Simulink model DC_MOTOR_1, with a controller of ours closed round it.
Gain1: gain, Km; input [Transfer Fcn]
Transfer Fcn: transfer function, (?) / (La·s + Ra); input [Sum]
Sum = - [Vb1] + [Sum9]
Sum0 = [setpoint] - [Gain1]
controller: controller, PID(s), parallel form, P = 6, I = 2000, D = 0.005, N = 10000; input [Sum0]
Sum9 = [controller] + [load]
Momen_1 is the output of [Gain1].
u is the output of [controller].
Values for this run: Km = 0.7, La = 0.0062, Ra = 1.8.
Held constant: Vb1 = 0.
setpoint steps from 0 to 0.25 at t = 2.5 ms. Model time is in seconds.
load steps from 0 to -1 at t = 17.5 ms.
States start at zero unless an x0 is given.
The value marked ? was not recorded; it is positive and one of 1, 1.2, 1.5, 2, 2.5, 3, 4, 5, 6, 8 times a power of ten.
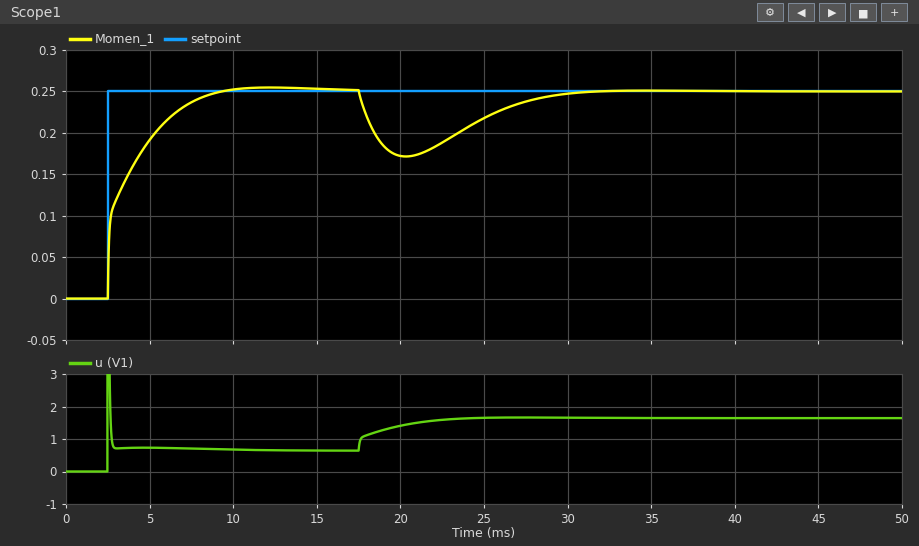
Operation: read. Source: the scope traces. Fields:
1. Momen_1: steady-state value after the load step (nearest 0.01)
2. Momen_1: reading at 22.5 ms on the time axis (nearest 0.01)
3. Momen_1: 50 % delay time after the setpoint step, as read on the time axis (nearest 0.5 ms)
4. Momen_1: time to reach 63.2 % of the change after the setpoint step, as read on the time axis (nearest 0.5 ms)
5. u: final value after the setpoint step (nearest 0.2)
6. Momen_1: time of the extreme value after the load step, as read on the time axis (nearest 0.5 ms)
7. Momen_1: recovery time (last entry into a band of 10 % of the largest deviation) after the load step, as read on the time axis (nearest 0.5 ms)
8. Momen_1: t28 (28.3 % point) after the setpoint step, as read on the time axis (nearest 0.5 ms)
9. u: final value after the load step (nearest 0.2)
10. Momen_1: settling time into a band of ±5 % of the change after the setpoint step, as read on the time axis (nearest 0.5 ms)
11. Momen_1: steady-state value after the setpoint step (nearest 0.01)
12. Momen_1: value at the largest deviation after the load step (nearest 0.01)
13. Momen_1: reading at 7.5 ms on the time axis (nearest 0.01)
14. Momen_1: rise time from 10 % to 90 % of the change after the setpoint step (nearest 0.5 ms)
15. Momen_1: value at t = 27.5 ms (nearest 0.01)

0.25
0.19
3.0 ms
4.0 ms
0.6
20.5 ms
28.5 ms
2.5 ms
1.6
7.5 ms
0.25
0.17
0.24
4.0 ms
0.24
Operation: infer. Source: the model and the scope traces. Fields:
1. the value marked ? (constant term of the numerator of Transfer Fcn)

1
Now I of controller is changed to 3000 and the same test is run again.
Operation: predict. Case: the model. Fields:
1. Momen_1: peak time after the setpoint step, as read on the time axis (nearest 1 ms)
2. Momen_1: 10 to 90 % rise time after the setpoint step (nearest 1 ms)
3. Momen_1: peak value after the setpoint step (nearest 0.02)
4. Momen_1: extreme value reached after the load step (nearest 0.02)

9 ms
3 ms
0.26
0.18
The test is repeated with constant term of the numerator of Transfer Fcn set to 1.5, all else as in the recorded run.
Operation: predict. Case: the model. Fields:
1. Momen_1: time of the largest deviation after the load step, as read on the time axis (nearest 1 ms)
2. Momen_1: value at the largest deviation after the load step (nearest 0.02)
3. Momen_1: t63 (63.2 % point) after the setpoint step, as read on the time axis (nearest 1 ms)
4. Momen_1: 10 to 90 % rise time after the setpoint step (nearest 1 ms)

20 ms
0.16
3 ms
3 ms
